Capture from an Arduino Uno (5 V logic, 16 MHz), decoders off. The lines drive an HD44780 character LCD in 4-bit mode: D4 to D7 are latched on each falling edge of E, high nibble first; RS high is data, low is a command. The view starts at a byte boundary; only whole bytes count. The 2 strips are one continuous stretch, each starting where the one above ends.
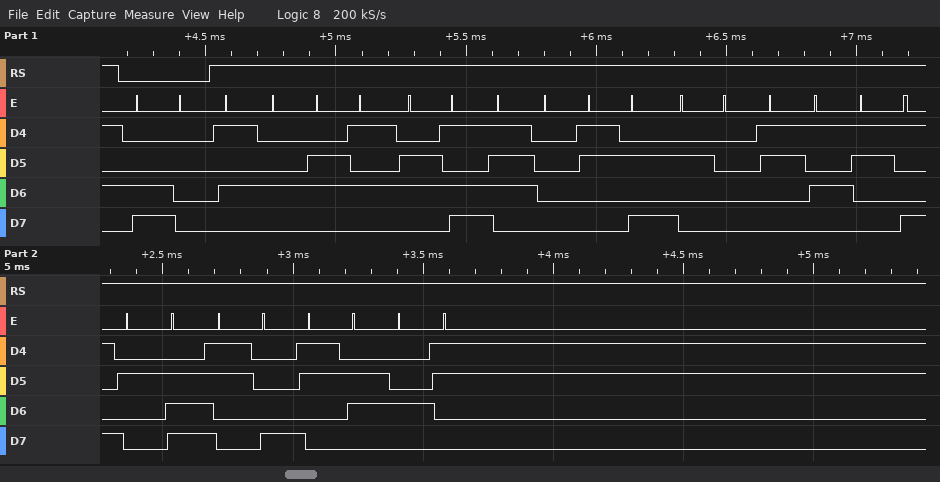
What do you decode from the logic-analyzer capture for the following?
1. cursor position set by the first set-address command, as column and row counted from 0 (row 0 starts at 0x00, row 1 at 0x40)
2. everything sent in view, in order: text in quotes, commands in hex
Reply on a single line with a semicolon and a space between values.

column 0, row 1; 0xC0 "Temp: 59.86C"
